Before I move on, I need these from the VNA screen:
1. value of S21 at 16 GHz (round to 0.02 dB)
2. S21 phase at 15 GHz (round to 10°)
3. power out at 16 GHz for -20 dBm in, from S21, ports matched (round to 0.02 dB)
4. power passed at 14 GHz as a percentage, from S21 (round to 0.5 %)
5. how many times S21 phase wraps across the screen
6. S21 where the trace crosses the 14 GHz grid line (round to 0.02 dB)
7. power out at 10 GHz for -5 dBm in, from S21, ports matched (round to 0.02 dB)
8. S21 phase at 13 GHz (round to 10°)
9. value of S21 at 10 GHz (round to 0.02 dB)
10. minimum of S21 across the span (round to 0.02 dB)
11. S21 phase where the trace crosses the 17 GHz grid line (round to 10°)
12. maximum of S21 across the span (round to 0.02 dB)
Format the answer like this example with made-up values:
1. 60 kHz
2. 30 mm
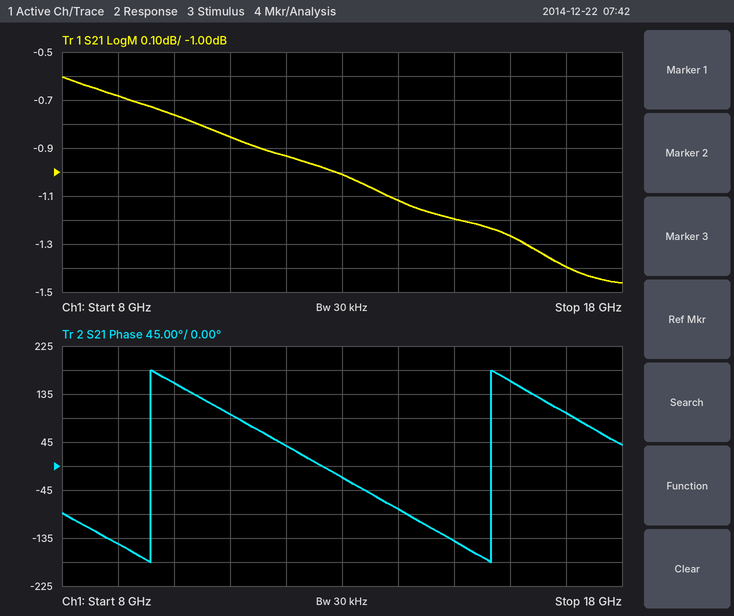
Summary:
1. -1.26 dB
2. -140°
3. -21.26 dBm
4. 77.5 %
5. 2
6. -1.12 dB
7. -5.76 dBm
8. -20°
9. -0.76 dB
10. -1.46 dB
11. 100°
12. -0.60 dB
